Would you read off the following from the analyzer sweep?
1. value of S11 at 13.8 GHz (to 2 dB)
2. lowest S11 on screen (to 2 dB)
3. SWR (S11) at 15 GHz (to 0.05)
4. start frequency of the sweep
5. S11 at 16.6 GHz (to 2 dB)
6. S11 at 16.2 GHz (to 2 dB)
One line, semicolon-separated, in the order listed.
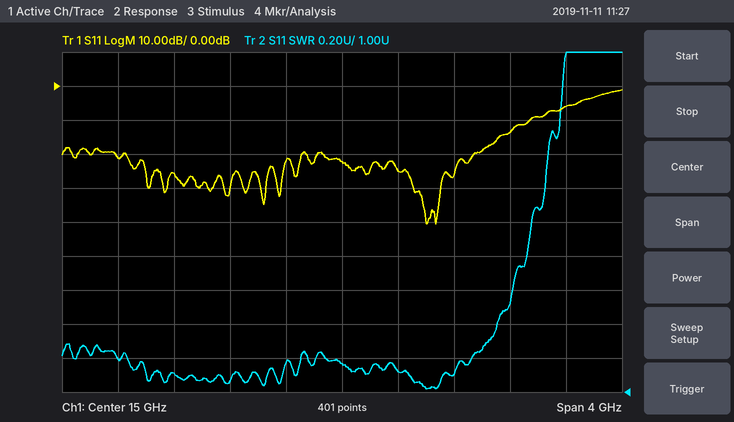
-26 dB; -40 dB; 1.15; 13 GHz; -6 dB; -14 dB
